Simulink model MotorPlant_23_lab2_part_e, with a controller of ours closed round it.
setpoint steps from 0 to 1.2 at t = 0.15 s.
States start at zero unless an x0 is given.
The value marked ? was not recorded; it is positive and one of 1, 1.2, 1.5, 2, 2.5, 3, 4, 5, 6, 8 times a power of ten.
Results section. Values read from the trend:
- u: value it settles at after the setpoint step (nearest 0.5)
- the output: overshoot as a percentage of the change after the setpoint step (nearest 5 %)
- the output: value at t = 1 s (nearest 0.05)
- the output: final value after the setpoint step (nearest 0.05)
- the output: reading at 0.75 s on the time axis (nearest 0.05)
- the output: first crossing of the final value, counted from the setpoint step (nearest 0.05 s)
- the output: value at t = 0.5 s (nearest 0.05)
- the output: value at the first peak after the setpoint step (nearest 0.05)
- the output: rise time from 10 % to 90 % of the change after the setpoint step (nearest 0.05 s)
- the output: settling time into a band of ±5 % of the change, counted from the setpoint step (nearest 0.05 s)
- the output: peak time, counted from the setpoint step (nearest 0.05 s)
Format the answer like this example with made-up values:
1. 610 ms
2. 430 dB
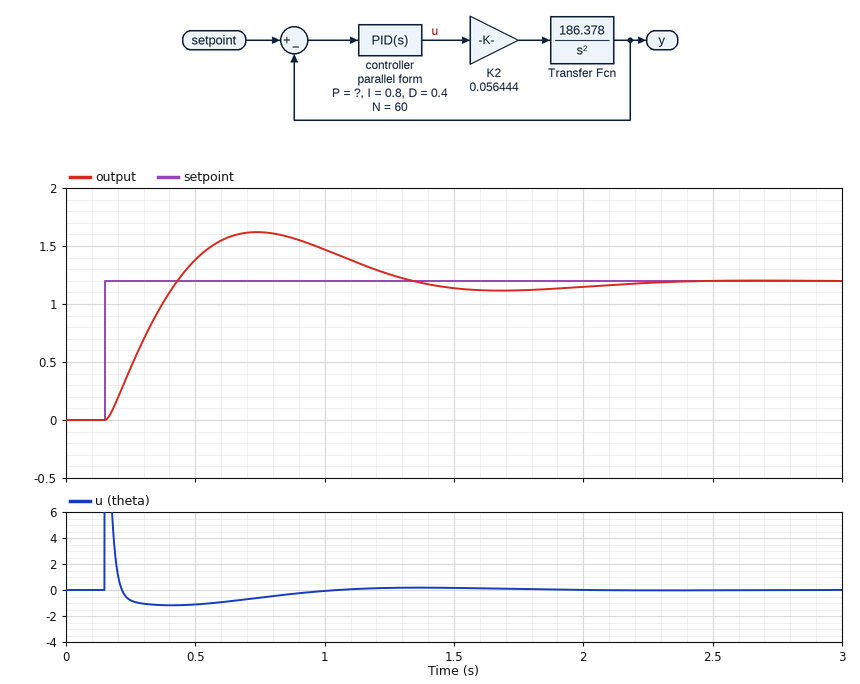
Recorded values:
1. 0.0
2. 35 %
3. 1.45
4. 1.20
5. 1.60
6. 0.30 s
7. 1.40
8. 1.60
9. 0.20 s
10. 1.80 s
11. 0.60 s
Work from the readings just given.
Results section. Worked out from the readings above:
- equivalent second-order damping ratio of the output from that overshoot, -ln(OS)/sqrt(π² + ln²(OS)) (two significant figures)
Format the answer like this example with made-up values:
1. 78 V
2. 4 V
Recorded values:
1. 0.32
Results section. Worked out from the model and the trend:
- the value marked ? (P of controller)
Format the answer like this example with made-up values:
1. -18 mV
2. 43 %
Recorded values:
1. 1.5
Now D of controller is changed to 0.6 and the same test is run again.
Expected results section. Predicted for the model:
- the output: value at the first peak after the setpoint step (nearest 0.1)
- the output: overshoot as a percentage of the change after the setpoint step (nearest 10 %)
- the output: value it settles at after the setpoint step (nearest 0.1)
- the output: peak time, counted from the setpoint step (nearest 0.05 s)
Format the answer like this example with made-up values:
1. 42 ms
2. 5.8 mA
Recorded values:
1. 1.5
2. 20 %
3. 1.2
4. 0.50 s
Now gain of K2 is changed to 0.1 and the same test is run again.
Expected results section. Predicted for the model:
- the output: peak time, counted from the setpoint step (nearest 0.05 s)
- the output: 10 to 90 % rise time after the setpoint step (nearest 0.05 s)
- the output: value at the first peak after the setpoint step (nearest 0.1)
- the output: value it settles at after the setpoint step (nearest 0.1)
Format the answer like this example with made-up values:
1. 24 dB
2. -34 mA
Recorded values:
1. 0.40 s
2. 0.15 s
3. 1.5
4. 1.2
